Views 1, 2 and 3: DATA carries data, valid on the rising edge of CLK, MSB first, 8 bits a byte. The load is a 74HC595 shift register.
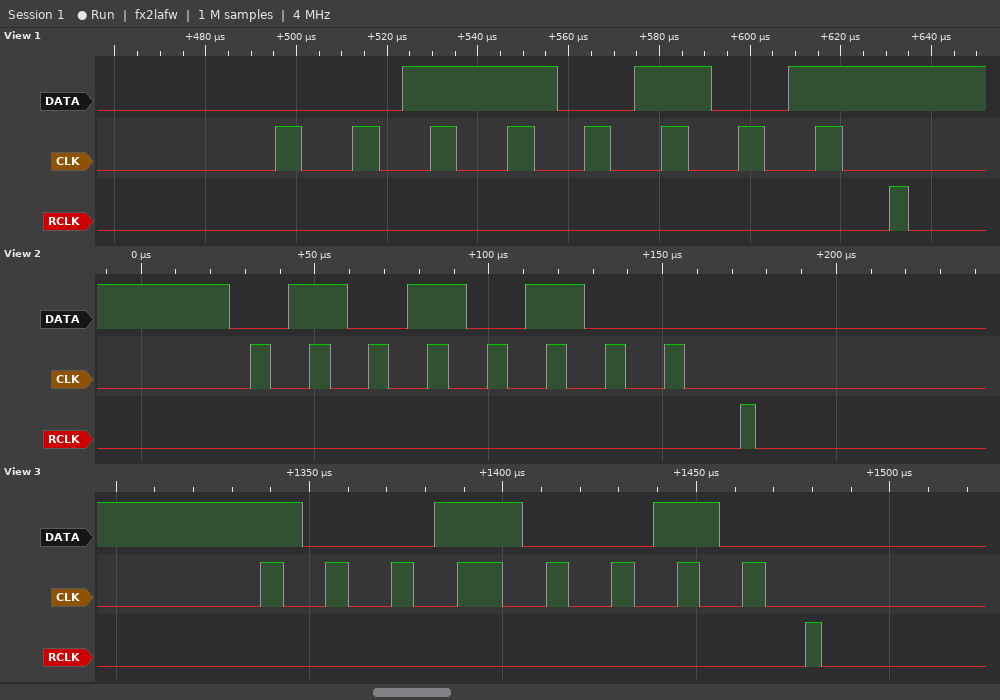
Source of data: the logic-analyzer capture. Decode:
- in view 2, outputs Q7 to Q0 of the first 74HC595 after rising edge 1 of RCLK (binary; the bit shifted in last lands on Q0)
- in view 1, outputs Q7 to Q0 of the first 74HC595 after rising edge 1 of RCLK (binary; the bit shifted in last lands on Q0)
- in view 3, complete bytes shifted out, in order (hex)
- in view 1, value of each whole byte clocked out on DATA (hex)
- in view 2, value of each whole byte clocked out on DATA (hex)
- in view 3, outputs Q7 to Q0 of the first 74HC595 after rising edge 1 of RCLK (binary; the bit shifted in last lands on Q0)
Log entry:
01010100
00110101
92
35
54
10010010
